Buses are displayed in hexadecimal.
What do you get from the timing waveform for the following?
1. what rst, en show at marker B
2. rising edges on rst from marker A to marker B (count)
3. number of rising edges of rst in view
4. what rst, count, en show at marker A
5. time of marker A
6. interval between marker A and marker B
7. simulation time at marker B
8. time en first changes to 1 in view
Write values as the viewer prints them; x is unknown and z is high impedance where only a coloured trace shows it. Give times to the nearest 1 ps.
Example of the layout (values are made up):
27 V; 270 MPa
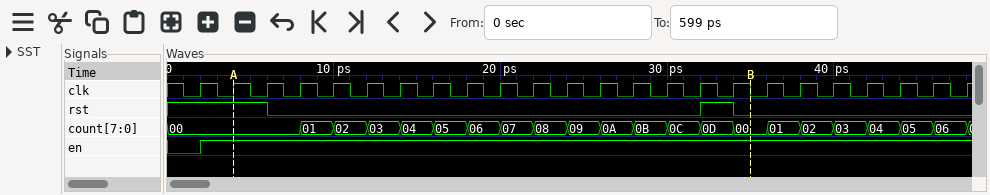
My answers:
rst=0, en=1; 1; 1; rst=1, count=00, en=1; 4 ps; 31 ps; 35 ps; 2 ps
